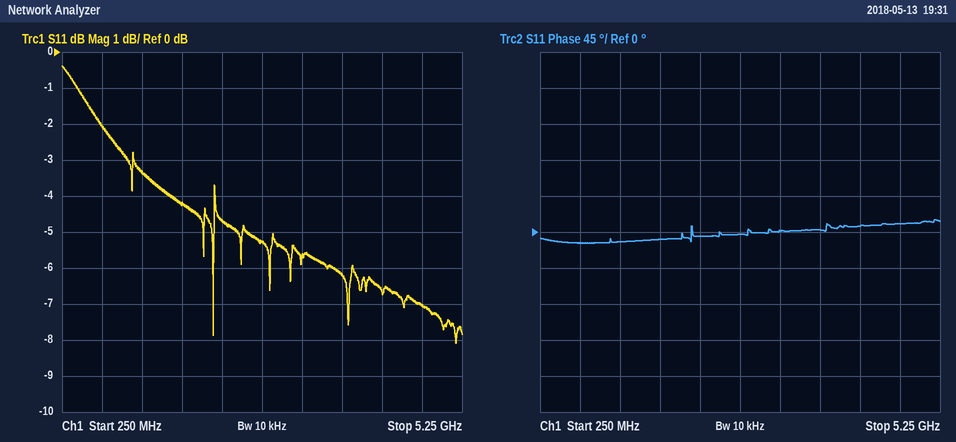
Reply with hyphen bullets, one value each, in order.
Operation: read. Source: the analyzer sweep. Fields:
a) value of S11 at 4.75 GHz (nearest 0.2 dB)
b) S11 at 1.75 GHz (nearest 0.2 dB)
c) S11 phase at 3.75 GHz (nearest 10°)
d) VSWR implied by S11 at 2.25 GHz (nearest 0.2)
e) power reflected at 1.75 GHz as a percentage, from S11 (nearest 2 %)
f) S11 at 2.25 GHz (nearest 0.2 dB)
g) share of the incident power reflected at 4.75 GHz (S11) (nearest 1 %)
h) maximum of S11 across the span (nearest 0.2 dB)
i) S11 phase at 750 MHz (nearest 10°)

- -7.0 dB
- -4.2 dB
- 0°
- 3.8
- 38 %
- -4.6 dB
- 20 %
- -0.4 dB
- -10°
